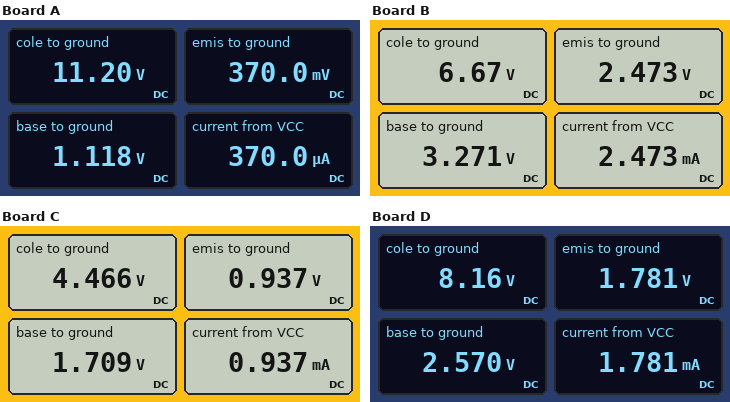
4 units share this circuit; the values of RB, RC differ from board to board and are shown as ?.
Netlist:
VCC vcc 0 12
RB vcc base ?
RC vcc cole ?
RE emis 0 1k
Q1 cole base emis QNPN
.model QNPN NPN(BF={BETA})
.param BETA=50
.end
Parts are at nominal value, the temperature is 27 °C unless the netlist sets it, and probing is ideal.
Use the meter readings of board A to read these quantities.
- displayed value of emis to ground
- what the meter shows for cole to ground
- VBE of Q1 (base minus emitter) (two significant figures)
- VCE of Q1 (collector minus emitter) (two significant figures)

370.0 mV
11.20 V
750 mV
11 V
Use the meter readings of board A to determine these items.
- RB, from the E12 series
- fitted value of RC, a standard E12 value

1.5 MΩ
2.2 kΩ
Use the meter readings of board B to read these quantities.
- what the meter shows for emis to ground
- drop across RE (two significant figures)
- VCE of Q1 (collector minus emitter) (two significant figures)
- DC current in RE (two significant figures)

2.473 V
2.5 V
4.2 V
2.5 mA
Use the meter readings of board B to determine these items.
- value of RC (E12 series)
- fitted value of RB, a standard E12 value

2.2 kΩ
180 kΩ
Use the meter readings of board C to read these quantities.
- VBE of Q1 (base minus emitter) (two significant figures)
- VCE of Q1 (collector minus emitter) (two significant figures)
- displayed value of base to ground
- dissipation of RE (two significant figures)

770 mV
3.5 V
1.709 V
880 µW
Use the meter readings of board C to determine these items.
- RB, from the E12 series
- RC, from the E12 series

560 kΩ
8.2 kΩ
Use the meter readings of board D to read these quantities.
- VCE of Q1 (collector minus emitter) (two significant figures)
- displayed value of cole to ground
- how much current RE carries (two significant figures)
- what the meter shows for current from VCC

6.4 V
8.16 V
1.8 mA
1.781 mA
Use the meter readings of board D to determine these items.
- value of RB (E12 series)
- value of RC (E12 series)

270 kΩ
2.2 kΩ
